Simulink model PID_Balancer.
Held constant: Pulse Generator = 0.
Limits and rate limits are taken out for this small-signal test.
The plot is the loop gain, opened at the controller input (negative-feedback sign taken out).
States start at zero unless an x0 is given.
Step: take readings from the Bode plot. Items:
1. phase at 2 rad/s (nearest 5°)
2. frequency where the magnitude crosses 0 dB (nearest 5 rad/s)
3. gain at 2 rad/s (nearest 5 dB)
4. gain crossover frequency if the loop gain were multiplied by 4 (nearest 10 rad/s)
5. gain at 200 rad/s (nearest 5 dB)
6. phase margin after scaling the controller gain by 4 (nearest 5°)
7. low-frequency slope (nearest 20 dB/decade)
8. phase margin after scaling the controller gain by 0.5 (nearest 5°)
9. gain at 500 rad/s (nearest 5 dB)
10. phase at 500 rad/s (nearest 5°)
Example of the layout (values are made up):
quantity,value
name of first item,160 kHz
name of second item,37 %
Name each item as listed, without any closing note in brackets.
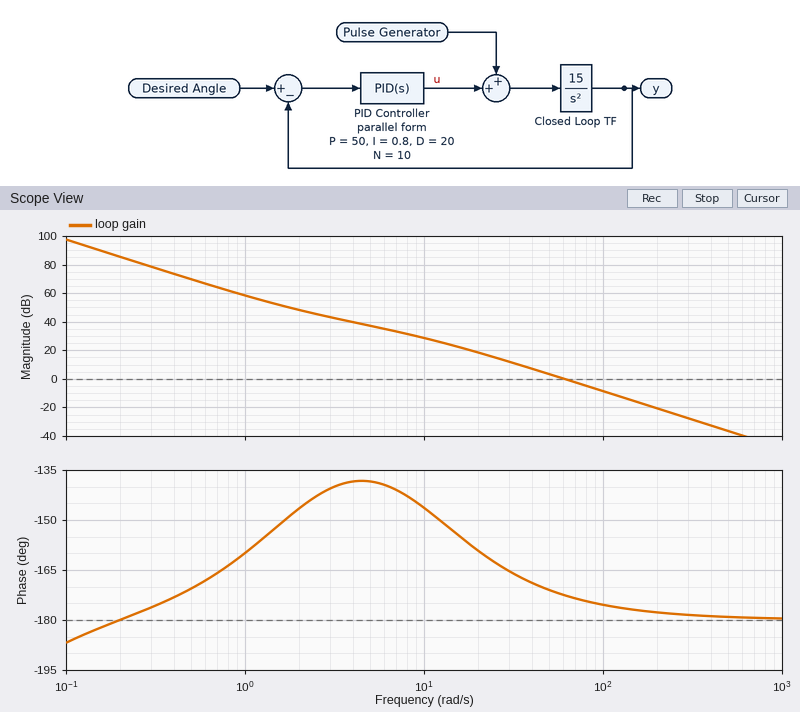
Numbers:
quantity,value
phase at 2 rad/s,-145°
frequency where the magnitude crosses 0 dB,60 rad/s
gain at 2 rad/s,50 dB
gain crossover frequency if the loop gain were multiplied by 4,120 rad/s
gain at 200 rad/s,-20 dB
phase margin after scaling the controller gain by 4,5°
low-frequency slope,-40 dB/decade
phase margin after scaling the controller gain by 0.5,10°
gain at 500 rad/s,-35 dB
phase at 500 rad/s,-180°
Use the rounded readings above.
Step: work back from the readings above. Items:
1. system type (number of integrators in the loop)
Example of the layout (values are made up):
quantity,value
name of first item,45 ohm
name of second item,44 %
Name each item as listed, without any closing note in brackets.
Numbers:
quantity,value
system type,2
